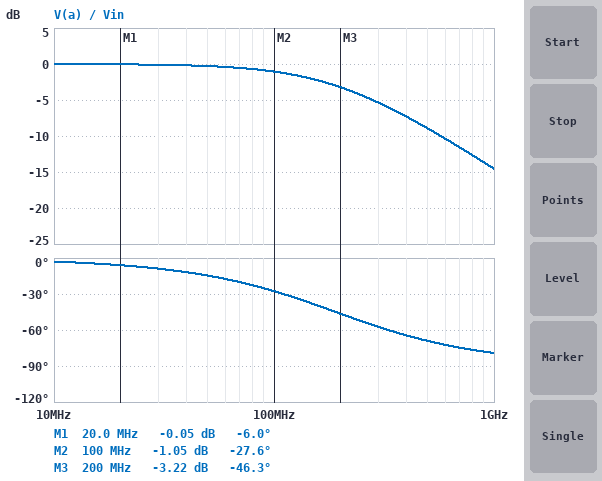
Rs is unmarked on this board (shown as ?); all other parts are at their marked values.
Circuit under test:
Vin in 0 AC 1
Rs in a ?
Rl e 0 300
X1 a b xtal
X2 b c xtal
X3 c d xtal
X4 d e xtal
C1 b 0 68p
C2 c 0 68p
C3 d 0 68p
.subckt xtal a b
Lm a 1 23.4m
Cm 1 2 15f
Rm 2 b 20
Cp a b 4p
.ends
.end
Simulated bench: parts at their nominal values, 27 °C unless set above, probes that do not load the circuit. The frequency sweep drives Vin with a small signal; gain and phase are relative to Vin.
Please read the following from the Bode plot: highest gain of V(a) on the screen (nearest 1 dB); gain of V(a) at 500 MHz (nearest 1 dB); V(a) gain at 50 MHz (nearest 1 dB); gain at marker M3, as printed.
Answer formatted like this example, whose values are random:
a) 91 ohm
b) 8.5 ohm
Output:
a) 0 dB
b) -9 dB
c) 0 dB
d) -3.22 dB
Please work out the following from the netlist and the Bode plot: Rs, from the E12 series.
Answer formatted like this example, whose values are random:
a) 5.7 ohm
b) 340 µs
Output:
a) 220 Ω
